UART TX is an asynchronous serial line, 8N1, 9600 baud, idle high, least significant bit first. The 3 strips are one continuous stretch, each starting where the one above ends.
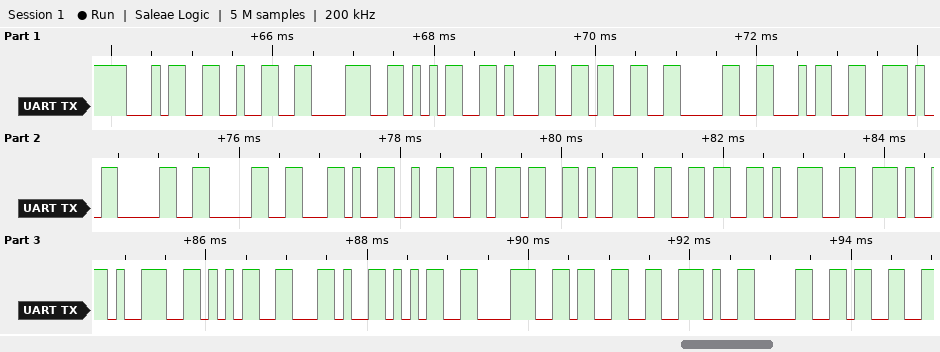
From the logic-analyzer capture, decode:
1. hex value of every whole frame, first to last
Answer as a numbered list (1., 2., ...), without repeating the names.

1. 34 32 38 35 31 33 30 34 2E 30 30 2C 32 37 39 36 39 2E 39 35 2C 35 38 33 2E 30 33
